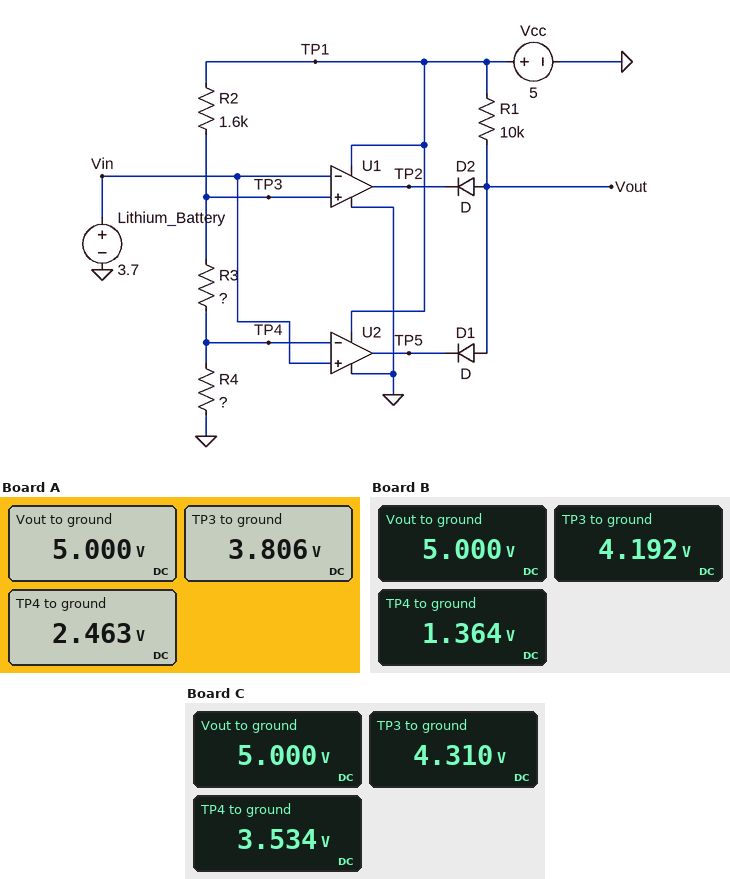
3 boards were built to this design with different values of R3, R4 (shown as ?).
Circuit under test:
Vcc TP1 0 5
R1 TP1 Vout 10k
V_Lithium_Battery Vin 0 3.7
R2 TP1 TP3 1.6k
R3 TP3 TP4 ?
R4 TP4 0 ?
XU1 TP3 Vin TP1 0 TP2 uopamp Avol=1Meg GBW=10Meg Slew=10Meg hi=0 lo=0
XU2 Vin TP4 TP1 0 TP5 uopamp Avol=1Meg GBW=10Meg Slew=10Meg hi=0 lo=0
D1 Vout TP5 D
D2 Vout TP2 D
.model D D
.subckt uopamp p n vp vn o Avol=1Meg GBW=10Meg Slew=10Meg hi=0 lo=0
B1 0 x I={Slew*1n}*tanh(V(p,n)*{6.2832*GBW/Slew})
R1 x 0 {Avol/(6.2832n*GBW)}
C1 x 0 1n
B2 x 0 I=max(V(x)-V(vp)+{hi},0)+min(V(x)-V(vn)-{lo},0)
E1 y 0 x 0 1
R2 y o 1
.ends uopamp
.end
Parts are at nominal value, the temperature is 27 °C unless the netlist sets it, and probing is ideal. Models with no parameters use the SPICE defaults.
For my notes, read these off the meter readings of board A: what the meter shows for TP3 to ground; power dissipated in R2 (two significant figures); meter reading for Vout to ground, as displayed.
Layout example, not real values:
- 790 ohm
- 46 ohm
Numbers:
- 3.806 V
- 890 µW
- 5.000 V
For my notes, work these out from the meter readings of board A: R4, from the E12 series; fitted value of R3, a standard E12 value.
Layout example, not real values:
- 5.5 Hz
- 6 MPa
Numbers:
- 3.3 kΩ
- 1.8 kΩ
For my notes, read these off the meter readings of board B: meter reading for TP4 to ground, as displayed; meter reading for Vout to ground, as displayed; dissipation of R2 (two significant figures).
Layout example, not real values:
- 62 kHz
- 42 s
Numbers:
- 1.364 V
- 5.000 V
- 410 µW
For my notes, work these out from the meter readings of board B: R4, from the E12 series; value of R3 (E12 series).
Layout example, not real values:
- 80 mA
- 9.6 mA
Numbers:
- 2.7 kΩ
- 5.6 kΩ
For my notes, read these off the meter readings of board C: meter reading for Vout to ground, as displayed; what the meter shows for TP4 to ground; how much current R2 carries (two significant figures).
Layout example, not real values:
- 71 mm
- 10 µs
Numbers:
- 5.000 V
- 3.534 V
- 430 µA
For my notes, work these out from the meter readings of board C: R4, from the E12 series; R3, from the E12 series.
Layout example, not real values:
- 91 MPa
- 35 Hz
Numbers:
- 8.2 kΩ
- 1.8 kΩ
